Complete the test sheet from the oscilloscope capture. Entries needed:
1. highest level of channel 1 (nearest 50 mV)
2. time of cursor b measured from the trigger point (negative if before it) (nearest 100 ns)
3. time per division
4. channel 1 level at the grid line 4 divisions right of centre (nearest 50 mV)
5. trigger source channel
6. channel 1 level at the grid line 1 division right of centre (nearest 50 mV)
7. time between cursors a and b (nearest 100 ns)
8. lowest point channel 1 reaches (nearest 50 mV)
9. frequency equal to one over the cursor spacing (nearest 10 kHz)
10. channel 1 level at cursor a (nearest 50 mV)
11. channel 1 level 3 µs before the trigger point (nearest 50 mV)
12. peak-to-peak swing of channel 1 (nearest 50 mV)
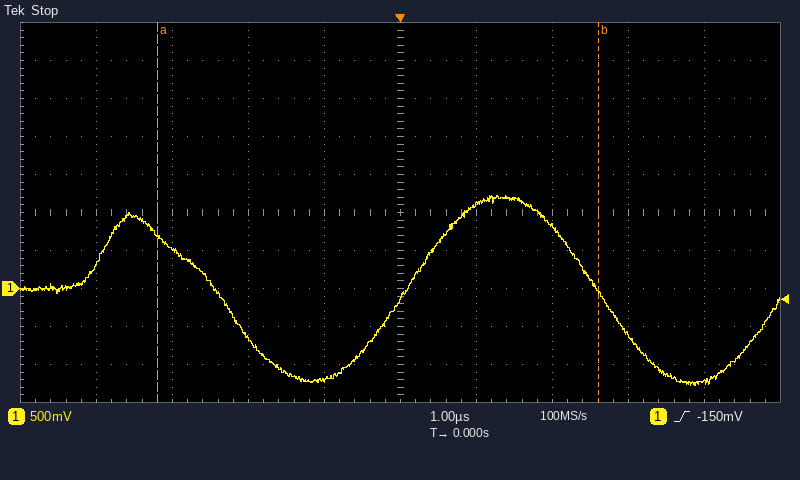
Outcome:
1.20 V
+2.6 µs
1 µs
-1.20 V
channel 1
1.10 V
5.8 µs
-1.30 V
170 kHz
700 mV
500 mV
2.50 V
